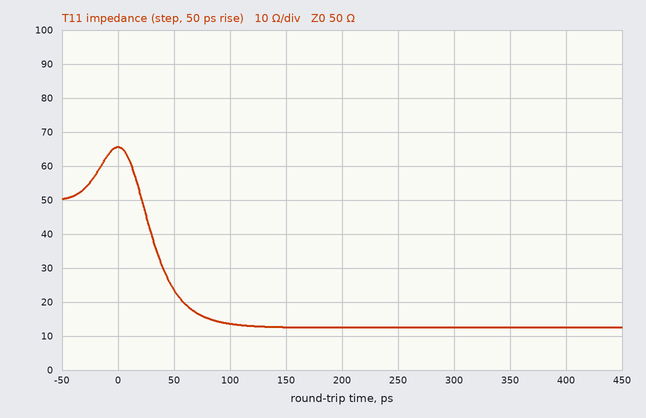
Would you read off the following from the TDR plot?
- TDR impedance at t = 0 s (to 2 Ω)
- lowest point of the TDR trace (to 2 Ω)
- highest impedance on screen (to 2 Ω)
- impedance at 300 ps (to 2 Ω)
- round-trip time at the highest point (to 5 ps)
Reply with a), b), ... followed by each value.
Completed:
a) 66 Ω
b) 12 Ω
c) 66 Ω
d) 12 Ω
e) 0 ps
